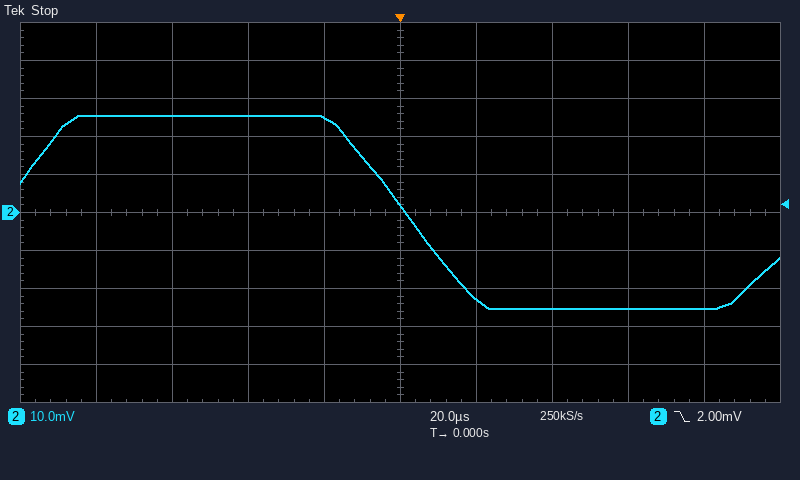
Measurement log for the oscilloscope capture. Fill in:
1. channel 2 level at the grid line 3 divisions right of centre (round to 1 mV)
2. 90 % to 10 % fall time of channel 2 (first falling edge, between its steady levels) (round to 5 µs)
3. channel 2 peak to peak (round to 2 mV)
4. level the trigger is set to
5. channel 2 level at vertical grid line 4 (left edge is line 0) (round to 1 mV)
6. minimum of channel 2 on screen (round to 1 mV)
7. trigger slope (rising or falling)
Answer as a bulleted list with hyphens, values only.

- -25 mV
- 30 µs
- 50 mV
- 2.00 mV
- 25 mV
- -25 mV
- falling
